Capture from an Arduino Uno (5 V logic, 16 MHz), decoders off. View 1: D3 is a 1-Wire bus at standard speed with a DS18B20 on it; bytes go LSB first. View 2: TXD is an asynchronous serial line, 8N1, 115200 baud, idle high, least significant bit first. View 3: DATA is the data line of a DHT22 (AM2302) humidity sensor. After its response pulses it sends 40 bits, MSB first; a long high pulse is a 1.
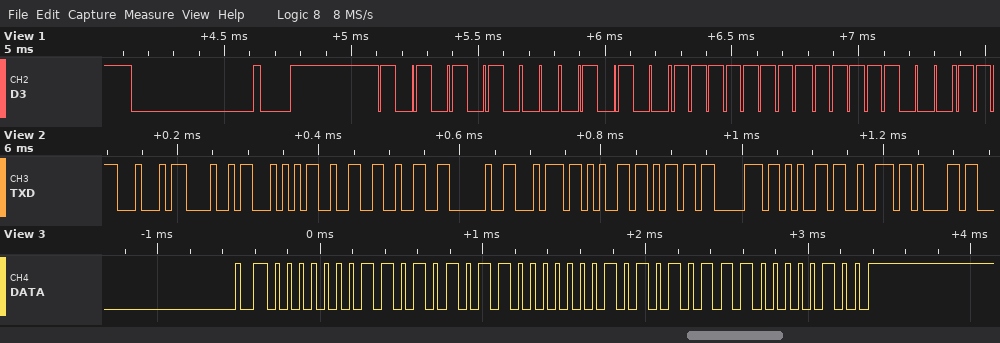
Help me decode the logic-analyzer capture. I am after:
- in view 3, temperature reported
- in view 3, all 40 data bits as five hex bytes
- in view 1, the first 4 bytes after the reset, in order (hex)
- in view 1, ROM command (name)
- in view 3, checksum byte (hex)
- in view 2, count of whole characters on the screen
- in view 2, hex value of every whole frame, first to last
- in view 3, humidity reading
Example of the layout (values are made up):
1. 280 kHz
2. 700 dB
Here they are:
1. 34.3 °C
2. 01 AB 01 57 04
3. 55 28 FF 1F
4. Match ROM
5. 0x04
6. 13
7. 44 48 54 32 32 20 74 65 6D 70 65 72 61
8. 42.7 %
